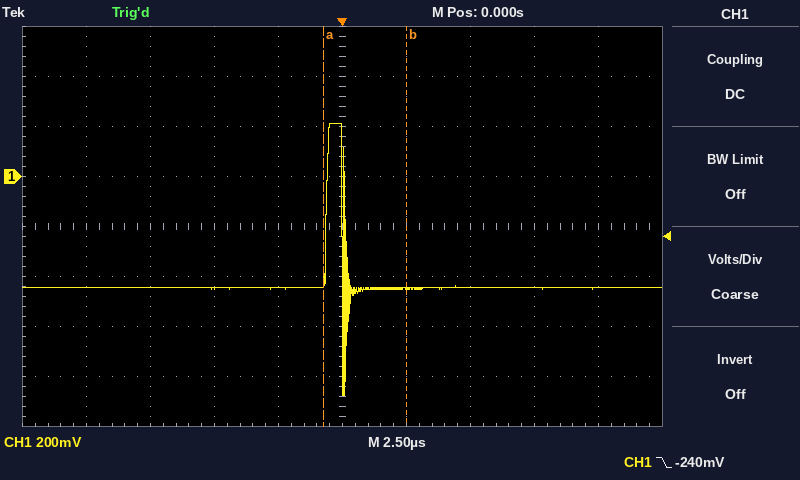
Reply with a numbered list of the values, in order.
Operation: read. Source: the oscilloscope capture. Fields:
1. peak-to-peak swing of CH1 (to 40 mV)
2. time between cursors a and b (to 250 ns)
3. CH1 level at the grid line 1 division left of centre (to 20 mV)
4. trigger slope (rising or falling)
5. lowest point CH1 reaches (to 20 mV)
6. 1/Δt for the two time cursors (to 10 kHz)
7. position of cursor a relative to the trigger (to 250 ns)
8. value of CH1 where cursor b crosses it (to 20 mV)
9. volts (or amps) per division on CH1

1. 1.08 V
2. 3.25 µs
3. -440 mV
4. falling
5. -880 mV
6. 310 kHz
7. -750 ns
8. -440 mV
9. 200 mV
